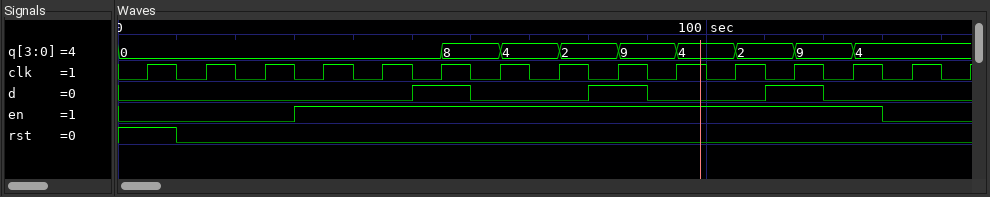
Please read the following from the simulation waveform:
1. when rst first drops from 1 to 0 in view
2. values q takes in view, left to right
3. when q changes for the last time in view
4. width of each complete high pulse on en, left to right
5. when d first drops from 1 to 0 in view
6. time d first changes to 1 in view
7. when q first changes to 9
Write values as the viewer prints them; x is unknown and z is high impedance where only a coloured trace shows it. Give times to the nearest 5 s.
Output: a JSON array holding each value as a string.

["10 s", "0, 8, 4, 2, 9, 4, 2, 9, 4", "125 s", "100 s", "60 s", "50 s", "85 s"]
